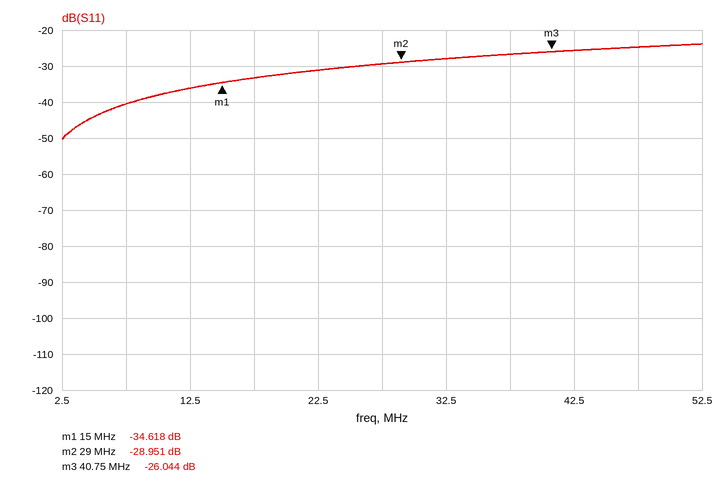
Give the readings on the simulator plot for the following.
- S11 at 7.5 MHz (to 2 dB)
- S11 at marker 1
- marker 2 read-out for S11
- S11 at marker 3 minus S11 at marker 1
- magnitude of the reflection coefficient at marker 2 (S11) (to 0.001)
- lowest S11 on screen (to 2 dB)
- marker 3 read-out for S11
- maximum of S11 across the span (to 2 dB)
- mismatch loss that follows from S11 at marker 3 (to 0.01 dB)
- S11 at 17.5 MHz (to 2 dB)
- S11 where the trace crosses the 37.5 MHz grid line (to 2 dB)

-40 dB
-34.618 dB
-28.951 dB
8.574 dB
0.036
-50 dB
-26.044 dB
-24 dB
0.01 dB
-34 dB
-26 dB
